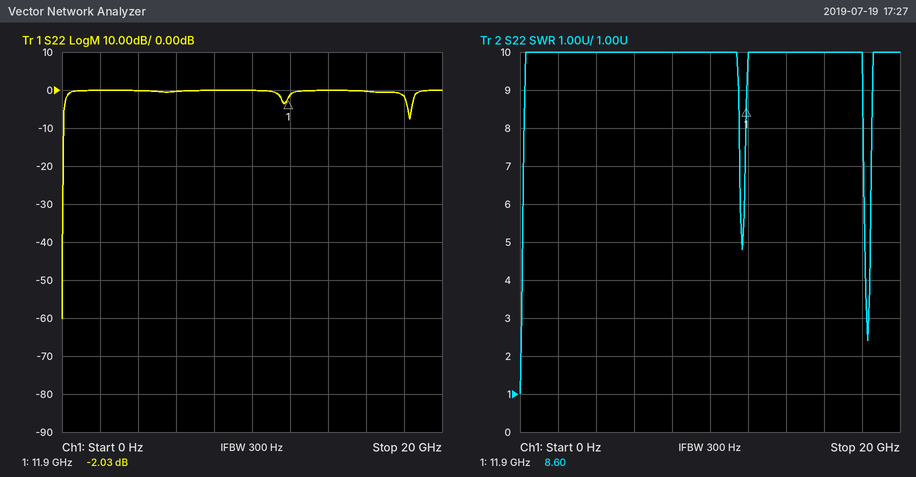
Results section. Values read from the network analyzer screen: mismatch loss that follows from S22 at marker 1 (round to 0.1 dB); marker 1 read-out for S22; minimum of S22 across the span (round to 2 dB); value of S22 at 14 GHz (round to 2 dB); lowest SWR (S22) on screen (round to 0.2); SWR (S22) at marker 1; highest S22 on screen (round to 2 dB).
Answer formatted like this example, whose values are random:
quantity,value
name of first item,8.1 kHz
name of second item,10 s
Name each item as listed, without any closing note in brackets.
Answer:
quantity,value
mismatch loss that follows from S22 at marker 1,4.3 dB
marker 1 read-out for S22,-2.03 dB
minimum of S22 across the span,-60 dB
value of S22 at 14 GHz,0 dB
lowest SWR (S22) on screen,1.0
SWR (S22) at marker 1,8.60
highest S22 on screen,0 dB
